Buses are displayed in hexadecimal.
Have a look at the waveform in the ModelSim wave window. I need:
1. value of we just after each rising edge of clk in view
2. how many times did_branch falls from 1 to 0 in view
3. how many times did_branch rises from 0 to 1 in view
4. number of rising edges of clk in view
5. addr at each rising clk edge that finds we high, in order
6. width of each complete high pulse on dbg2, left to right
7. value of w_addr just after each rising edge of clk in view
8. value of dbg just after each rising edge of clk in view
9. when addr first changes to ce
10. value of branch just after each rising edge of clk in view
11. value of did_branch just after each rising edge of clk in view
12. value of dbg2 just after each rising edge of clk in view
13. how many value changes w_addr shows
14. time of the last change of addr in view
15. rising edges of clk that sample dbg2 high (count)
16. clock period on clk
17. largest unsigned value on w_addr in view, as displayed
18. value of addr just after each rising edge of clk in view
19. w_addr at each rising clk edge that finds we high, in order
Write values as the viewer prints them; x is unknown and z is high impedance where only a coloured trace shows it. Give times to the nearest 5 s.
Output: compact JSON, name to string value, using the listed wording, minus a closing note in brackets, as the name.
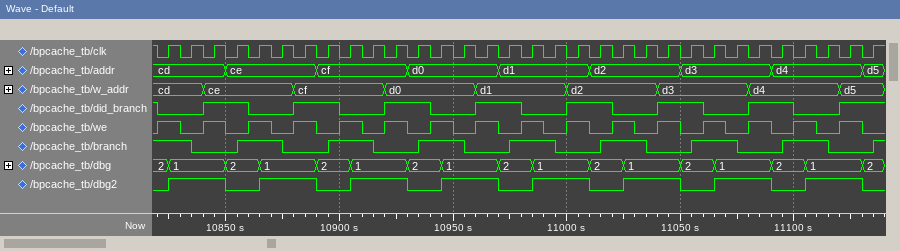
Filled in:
{"value of we just after each rising edge of clk in view": "1 0 1 0 1 0 1 0 1 0 1 0 1 0 1 0 1 0 1 0 1 0 1 0 1 0 1 0 1 0 1 0", "how many times did_branch falls from 1 to 0 in view": "8", "how many times did_branch rises from 0 to 1 in view": "8", "number of rising edges of clk in view": "32", "addr at each rising clk edge that finds we high, in order": "cd, cd, ce, ce, cf, cf, d0, d0, d1, d1, d2, d2, d3, d3, d4, d4", "width of each complete high pulse on dbg2, left to right": "25 s, 25 s, 25 s, 25 s, 25 s, 25 s, 25 s, 25 s", "value of w_addr just after each rising edge of clk in view": "cd, cd, ce, ce, ce, ce, cf, cf, cf, cf, d0, d0, d0, d0, d1, d1, d1, d1, d2, d2, d2, d2, d3, d3, d3, d3, d4, d4, d4, d4, d5, d5", "value of dbg just after each rising edge of clk in view": "1, 1, 1, 2, 1, 1, 1, 2, 1, 1, 1, 2, 1, 1, 1, 2, 1, 1, 1, 2, 1, 1, 1, 2, 1, 1, 1, 2, 1, 1, 1, 2", "when addr first changes to ce": "10850 s", "value of branch just after each rising edge of clk in view": "1 0 0 1 1 0 0 1 1 0 0 1 1 0 0 1 1 0 0 1 1 0 0 1 1 0 0 1 1 0 0 1", "value of did_branch just after each rising edge of clk in view": "0 0 1 1 0 0 1 1 0 0 1 1 0 0 1 1 0 0 1 1 0 0 1 1 0 0 1 1 0 0 1 1", "value of dbg2 just after each rising edge of clk in view": "1 1 1 0 1 1 1 0 1 1 1 0 1 1 1 0 1 1 1 0 1 1 1 0 1 1 1 0 1 1 1 0", "how many value changes w_addr shows": "8", "time of the last change of addr in view": "11130 s", "rising edges of clk that sample dbg2 high": "16", "clock period on clk": "10 s", "largest unsigned value on w_addr in view, as displayed": "d5", "value of addr just after each rising edge of clk in view": "cd, cd, cd, ce, ce, ce, ce, cf, cf, cf, cf, d0, d0, d0, d0, d1, d1, d1, d1, d2, d2, d2, d2, d3, d3, d3, d3, d4, d4, d4, d4, d5", "w_addr at each rising clk edge that finds we high, in order": "cd, ce, ce, cf, cf, d0, d0, d1, d1, d2, d2, d3, d3, d4, d4, d5"}
